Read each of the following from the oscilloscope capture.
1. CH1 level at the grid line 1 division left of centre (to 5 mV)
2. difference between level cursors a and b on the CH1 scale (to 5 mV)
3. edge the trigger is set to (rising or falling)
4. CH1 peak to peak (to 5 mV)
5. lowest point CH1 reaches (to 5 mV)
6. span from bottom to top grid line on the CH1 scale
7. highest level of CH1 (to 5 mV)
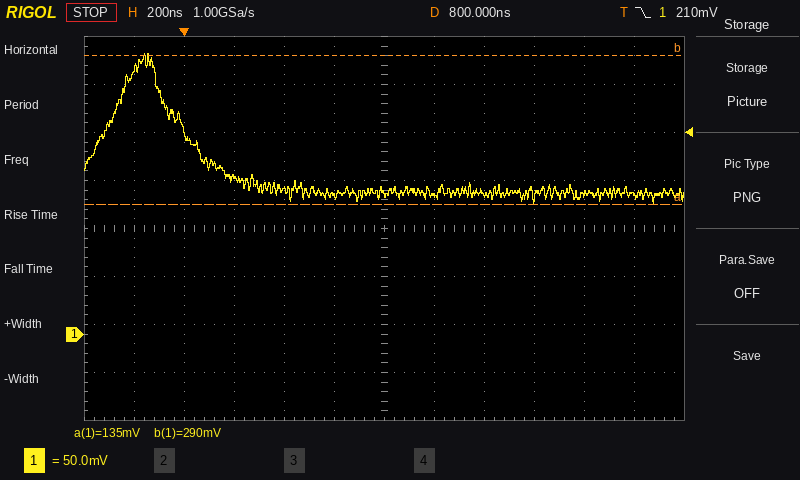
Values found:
145 mV
155 mV
falling
155 mV
135 mV
400 mV
290 mV
